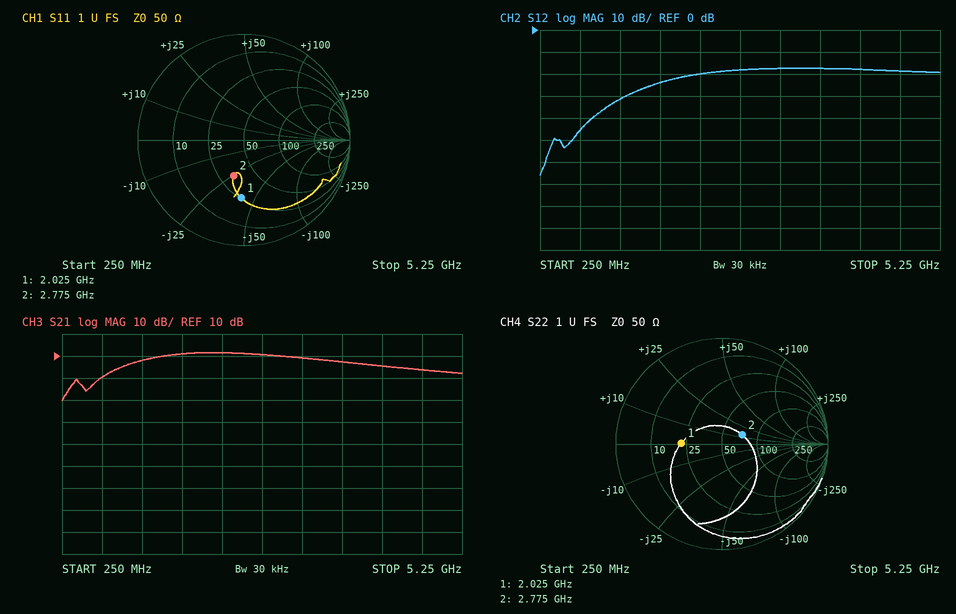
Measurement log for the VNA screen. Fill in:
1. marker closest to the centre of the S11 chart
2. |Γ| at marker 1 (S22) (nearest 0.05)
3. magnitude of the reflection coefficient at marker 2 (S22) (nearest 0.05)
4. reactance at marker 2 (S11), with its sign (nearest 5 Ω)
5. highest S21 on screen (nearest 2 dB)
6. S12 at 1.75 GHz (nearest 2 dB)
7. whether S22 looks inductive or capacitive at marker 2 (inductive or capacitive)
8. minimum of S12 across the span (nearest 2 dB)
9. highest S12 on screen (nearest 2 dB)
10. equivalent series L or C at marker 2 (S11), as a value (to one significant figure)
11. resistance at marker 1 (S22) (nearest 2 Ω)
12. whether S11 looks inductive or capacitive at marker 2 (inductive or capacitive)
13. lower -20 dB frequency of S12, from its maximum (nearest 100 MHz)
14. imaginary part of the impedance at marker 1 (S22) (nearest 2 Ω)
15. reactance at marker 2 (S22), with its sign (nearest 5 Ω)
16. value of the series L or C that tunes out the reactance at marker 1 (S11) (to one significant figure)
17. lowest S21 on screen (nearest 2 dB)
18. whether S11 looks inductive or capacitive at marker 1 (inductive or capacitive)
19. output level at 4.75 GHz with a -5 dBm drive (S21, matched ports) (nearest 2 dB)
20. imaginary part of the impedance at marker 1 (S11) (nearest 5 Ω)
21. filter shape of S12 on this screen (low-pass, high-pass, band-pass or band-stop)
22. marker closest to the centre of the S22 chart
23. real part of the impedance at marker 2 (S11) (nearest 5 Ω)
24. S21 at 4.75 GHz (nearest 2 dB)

marker 2
0.40
0.20
-25 Ω
12 dB
-24 dB
inductive
-66 dB
-18 dB
2 pF
22 Ω
capacitive
1.0 GHz
0 Ω
+15 Ω
3 nH
-10 dB
capacitive
-2 dBm
-40 Ω
high-pass
marker 2
35 Ω
4 dB
